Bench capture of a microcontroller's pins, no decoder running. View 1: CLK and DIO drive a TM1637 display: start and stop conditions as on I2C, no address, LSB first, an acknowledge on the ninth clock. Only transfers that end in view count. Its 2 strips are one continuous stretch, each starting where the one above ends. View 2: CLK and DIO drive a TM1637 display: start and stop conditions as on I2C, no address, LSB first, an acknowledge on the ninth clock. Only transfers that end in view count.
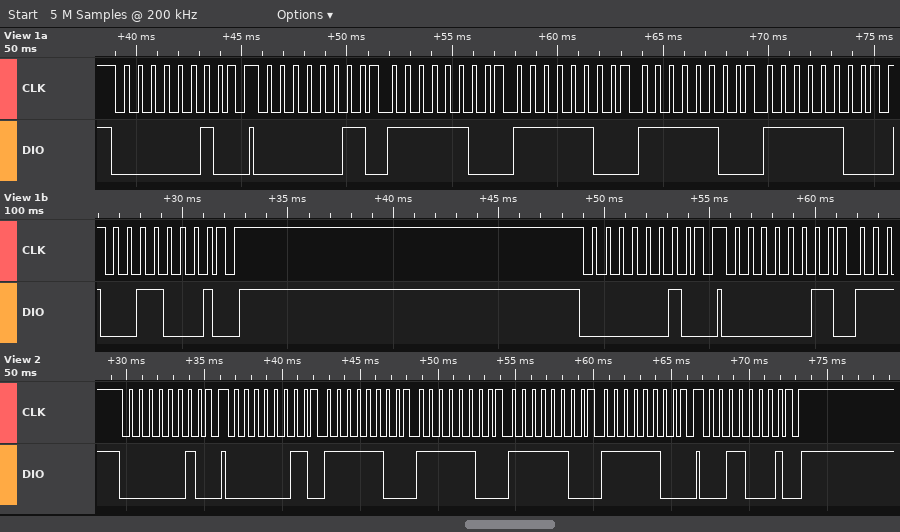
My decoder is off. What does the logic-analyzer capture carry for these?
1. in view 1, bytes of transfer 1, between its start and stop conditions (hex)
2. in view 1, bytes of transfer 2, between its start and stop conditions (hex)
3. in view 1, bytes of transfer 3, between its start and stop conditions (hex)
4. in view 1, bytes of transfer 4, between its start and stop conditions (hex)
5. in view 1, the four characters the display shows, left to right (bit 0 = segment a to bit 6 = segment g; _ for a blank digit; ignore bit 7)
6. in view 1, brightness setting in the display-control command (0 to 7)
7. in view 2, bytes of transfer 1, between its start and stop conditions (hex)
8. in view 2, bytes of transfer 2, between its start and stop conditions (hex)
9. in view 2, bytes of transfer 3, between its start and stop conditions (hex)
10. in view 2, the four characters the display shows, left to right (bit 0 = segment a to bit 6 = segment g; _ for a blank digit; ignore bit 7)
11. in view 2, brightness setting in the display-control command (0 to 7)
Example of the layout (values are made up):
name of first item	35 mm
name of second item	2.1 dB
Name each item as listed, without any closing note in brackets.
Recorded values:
in view 1, bytes of transfer 1, between its start and stop conditions	40
in view 1, bytes of transfer 2, between its start and stop conditions	C0 3F 3F 3F 3F
in view 1, bytes of transfer 3, between its start and stop conditions	8C
in view 1, bytes of transfer 4, between its start and stop conditions	40
in view 1, the four characters the display shows, left to right	0000
in view 1, brightness setting in the display-control command	4
in view 2, bytes of transfer 1, between its start and stop conditions	40
in view 2, bytes of transfer 2, between its start and stop conditions	C0 3F 3F 3F 3F
in view 2, bytes of transfer 3, between its start and stop conditions	8C
in view 2, the four characters the display shows, left to right	0000
in view 2, brightness setting in the display-control command	4
